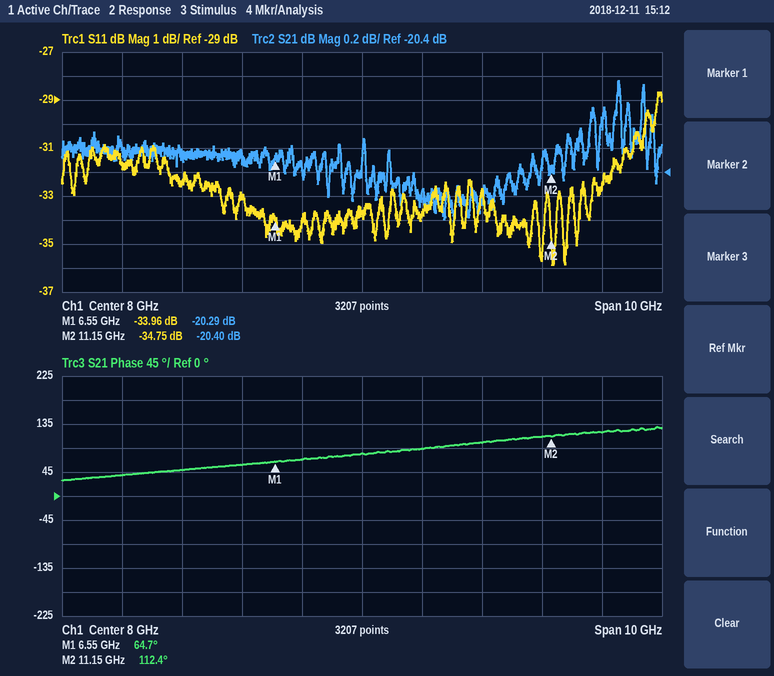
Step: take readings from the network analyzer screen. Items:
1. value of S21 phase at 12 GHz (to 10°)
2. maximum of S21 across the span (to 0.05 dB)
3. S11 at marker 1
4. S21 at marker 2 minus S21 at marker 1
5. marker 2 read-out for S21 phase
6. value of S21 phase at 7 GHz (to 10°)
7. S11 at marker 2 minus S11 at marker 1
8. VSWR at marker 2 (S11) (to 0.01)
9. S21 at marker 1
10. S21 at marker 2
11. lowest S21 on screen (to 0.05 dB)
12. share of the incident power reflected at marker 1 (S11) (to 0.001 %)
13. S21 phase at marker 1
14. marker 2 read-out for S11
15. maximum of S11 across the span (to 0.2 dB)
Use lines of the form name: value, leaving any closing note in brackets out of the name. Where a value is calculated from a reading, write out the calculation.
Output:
value of S21 phase at 12 GHz: 120°
maximum of S21 across the span: -19.65 dB
S11 at marker 1: -33.96 dB
S21 at marker 2 minus S21 at marker 1: -20.4 − (-20.29) = -0.11 dB
marker 2 read-out for S21 phase: 112.4°
value of S21 phase at 7 GHz: 70°
S11 at marker 2 minus S11 at marker 1: -34.75 − (-33.96) = -0.79 dB
VSWR at marker 2 (S11): (1 + 0.0183)/(1 − 0.0183) ≈ 1.04
S21 at marker 1: -20.29 dB
S21 at marker 2: -20.40 dB
lowest S21 on screen: -20.80 dB
share of the incident power reflected at marker 1 (S11): 10^(-33.96/10) ≈ 0.040 %
S21 phase at marker 1: 64.7°
marker 2 read-out for S11: -34.75 dB
maximum of S11 across the span: -28.6 dB
